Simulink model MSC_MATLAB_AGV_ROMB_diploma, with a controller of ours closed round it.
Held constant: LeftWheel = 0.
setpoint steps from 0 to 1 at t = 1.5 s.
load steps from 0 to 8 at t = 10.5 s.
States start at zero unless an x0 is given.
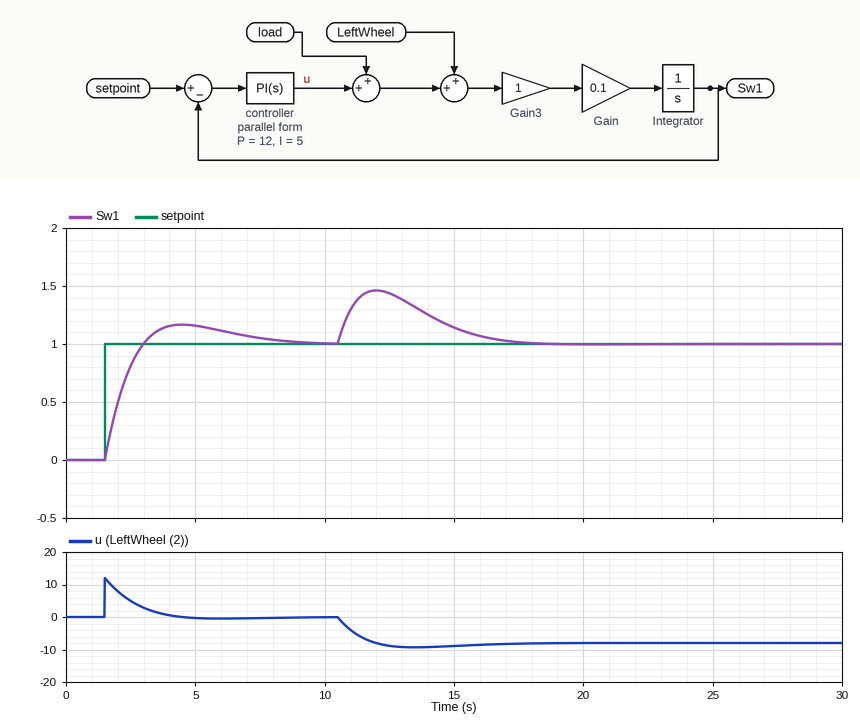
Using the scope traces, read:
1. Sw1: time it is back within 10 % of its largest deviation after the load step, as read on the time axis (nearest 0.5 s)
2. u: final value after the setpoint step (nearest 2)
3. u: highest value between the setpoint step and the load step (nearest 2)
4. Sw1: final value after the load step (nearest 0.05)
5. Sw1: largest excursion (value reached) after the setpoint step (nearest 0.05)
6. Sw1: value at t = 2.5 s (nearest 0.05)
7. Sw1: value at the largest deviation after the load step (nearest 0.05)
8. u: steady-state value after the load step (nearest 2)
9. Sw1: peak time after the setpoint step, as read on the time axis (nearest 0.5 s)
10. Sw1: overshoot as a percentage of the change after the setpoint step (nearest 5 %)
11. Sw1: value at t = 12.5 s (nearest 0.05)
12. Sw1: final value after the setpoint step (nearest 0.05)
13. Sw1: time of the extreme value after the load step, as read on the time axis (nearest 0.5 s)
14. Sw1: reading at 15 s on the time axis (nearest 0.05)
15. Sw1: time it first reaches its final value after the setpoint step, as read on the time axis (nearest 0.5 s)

16.5 s
0
12
1.00
1.15
0.80
1.45
-8
4.5 s
15 %
1.45
1.00
12.0 s
1.15
3.0 s
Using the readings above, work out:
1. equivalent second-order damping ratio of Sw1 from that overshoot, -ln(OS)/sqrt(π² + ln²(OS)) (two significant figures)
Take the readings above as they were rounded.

0.52
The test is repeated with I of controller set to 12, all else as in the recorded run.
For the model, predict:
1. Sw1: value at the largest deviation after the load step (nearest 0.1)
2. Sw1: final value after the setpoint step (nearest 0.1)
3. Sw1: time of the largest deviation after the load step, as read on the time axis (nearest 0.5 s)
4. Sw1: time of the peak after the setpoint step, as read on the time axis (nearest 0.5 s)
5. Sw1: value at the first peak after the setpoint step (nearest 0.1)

1.4
1.0
11.5 s
3.5 s
1.3
